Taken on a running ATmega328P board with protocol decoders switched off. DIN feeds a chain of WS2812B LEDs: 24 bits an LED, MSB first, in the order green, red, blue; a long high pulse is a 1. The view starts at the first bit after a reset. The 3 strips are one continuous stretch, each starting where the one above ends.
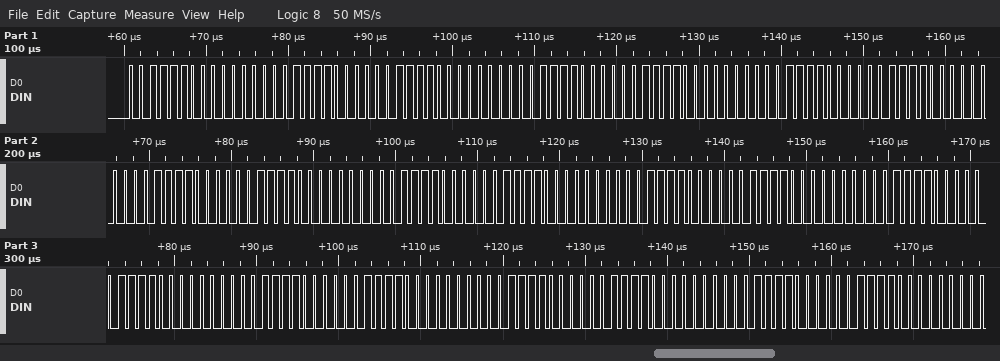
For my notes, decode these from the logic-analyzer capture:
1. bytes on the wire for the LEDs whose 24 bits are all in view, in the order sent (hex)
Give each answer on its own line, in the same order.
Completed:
3C 00 F0 3C 00 F0 3C 00 F0 3C 00 F0 3C 00 F0 3C 00 F0 3C 00 F0 3C 00 F0 3C 00 F0 3C 00 F0
